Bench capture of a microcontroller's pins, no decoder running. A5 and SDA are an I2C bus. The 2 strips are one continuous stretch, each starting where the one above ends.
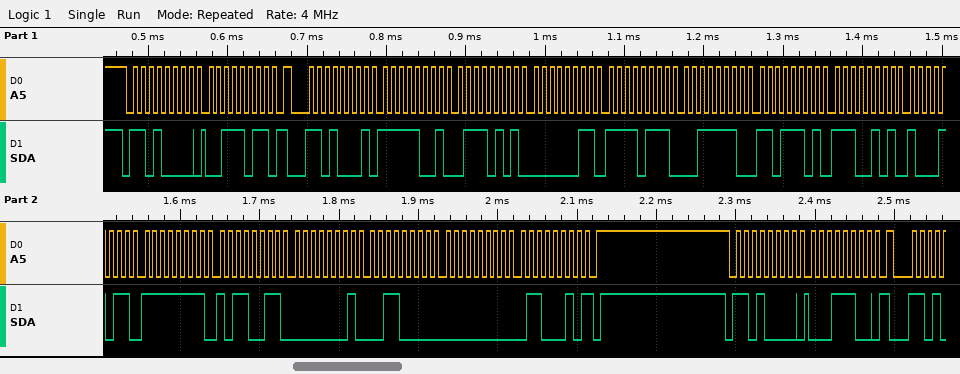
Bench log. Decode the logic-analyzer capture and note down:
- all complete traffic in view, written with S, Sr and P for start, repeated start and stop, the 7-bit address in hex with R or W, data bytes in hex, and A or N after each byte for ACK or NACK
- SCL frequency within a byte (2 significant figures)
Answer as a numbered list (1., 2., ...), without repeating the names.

1. S 68W A 3B A Sr 68R A F9 A 75 A 03 A F7 A 3E A DD A E5 A 8B A FF A B3 A 01 A 30 A 00 A 62 N P S 68W A 1C A
2. 100 kHz
